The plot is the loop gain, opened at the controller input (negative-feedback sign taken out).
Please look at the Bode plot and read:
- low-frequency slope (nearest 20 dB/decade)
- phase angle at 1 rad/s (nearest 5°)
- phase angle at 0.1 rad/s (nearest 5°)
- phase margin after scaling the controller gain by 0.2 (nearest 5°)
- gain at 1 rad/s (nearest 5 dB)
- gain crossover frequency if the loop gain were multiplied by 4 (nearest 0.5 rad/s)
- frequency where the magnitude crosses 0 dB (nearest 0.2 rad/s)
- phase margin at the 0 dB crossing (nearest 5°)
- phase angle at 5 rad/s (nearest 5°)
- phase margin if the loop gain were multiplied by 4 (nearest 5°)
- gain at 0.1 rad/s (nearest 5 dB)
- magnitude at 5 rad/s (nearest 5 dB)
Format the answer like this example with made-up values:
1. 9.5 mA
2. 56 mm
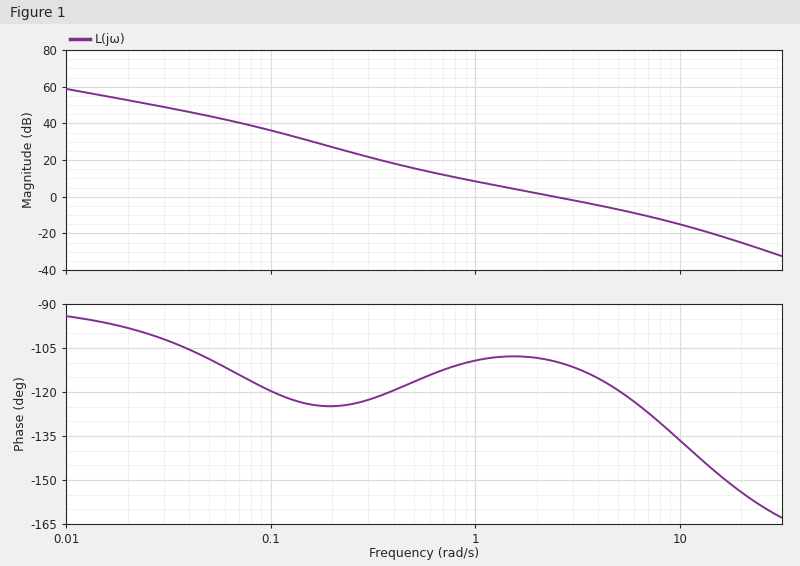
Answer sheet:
1. -20 dB/decade
2. -110°
3. -120°
4. 65°
5. 10 dB
6. 8.0 rad/s
7. 2.4 rad/s
8. 70°
9. -120°
10. 50°
11. 35 dB
12. -5 dB
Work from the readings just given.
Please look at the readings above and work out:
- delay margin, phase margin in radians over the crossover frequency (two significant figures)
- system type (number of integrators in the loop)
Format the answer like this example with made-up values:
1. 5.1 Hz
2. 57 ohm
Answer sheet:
1. 0.51 s
2. 1
